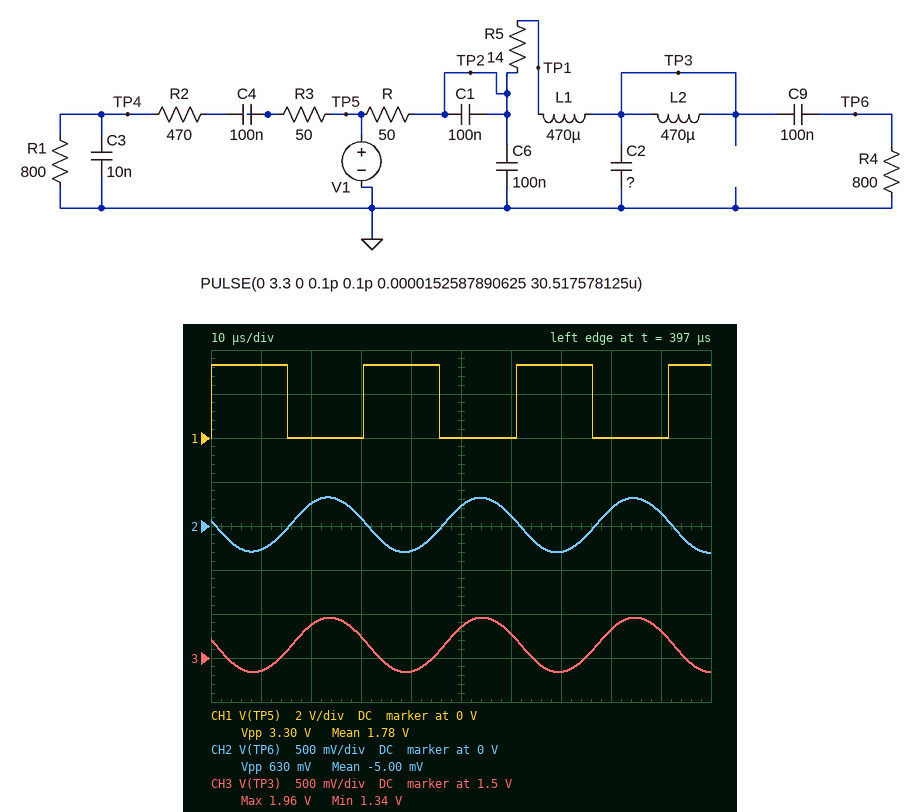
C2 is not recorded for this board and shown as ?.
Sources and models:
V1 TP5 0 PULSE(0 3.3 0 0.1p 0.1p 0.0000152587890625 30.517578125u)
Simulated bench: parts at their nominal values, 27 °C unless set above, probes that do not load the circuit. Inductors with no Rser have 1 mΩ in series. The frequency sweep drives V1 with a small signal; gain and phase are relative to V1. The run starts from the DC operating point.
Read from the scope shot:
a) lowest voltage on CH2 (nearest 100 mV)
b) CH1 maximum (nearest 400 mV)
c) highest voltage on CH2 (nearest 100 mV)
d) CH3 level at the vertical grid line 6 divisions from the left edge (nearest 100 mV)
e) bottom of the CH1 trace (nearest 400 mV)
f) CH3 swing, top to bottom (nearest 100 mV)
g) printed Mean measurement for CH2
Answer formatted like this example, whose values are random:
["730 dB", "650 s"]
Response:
["-300 mV", "3.2 V", "300 mV", "1.8 V", "0 V", "600 mV", "-5.00 mV"]
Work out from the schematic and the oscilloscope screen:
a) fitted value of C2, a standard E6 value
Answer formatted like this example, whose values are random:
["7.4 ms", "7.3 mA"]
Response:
["330 nF"]
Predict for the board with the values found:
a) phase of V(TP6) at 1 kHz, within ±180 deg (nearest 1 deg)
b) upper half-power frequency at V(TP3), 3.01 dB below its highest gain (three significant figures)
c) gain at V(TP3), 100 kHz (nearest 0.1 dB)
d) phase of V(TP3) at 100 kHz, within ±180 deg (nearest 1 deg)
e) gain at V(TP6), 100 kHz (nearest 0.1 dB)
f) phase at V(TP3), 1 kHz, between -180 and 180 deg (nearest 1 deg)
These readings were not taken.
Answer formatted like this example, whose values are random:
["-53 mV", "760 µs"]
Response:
["52 deg", "8.17 kHz", "-45.5 dB", "112 deg", "-45.5 dB", "-11 deg"]
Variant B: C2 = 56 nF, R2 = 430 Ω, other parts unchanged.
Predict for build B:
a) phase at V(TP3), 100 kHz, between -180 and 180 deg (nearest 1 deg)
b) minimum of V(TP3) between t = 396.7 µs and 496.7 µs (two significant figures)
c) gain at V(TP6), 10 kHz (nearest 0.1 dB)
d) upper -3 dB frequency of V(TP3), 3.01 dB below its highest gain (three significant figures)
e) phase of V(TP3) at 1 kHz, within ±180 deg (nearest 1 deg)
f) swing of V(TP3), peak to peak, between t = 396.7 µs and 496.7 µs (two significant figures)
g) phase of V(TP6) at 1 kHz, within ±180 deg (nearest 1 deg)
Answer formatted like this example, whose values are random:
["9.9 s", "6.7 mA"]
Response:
["114 deg", "-900 mV", "-0.9 dB", "41.2 kHz", "-5 deg", "5.1 V", "58 deg"]
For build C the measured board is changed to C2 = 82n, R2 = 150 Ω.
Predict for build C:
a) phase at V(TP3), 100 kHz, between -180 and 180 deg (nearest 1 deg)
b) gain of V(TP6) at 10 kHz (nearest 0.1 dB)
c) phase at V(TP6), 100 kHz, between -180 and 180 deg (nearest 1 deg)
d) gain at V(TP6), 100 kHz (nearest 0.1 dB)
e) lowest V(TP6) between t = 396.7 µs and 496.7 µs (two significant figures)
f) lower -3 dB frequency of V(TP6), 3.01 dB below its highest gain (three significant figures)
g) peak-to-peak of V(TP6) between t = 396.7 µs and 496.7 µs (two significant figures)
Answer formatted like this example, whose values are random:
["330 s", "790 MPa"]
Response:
["113 deg", "-1.0 dB", "114 deg", "-33.0 dB", "-1.9 V", "2.46 kHz", "3.9 V"]
